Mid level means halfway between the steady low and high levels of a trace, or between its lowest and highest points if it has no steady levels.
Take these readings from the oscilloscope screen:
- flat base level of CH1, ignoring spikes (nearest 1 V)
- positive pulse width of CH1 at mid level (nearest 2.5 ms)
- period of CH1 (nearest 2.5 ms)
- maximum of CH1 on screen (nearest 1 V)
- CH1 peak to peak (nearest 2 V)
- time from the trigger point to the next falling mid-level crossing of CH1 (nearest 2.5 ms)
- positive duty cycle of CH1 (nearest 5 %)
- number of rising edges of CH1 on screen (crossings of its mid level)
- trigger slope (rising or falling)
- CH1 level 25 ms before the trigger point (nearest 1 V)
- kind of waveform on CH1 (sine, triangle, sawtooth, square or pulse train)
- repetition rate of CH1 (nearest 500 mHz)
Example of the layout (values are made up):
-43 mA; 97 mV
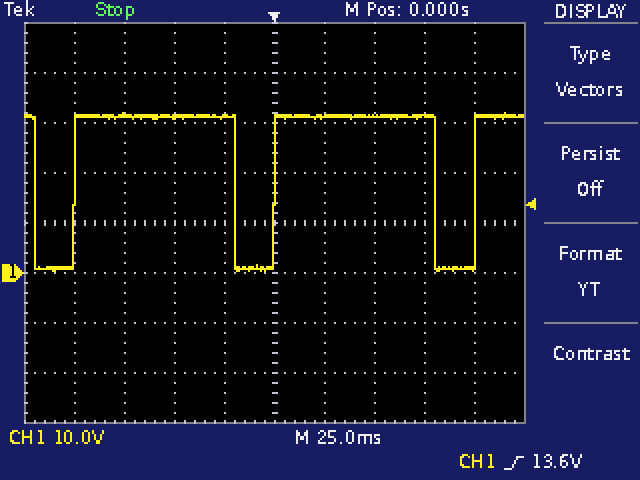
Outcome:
1 V; 80.0 ms; 100.0 ms; 32 V; 32 V; 80.0 ms; 80 %; 3; rising; 31 V; pulse train; 10.0 Hz
